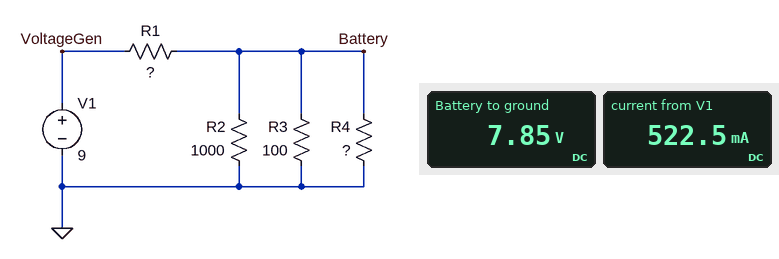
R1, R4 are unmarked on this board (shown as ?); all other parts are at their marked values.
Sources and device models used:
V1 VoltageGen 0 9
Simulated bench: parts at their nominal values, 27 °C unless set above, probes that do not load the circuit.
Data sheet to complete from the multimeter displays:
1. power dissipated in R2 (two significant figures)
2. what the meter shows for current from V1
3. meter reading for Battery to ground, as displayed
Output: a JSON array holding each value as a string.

["62 mW", "522.5 mA", "7.85 V"]
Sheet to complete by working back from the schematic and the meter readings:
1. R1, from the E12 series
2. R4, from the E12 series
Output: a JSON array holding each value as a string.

["2.2 Ω", "18 Ω"]
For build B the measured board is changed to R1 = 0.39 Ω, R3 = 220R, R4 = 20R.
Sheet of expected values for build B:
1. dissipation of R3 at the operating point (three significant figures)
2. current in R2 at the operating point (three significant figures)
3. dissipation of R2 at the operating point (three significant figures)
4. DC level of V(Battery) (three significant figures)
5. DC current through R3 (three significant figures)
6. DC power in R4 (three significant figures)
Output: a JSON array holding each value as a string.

["353 mW", "8.81 mA", "77.6 mW", "8.81 V", "40.0 mA", "3.88 W"]
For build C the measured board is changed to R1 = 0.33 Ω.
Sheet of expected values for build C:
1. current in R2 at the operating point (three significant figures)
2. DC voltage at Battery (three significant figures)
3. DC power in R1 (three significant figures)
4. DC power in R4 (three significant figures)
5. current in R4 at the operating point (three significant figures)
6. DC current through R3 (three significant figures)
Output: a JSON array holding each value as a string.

["8.81 mA", "8.81 V", "113 mW", "4.31 W", "489 mA", "88.1 mA"]
